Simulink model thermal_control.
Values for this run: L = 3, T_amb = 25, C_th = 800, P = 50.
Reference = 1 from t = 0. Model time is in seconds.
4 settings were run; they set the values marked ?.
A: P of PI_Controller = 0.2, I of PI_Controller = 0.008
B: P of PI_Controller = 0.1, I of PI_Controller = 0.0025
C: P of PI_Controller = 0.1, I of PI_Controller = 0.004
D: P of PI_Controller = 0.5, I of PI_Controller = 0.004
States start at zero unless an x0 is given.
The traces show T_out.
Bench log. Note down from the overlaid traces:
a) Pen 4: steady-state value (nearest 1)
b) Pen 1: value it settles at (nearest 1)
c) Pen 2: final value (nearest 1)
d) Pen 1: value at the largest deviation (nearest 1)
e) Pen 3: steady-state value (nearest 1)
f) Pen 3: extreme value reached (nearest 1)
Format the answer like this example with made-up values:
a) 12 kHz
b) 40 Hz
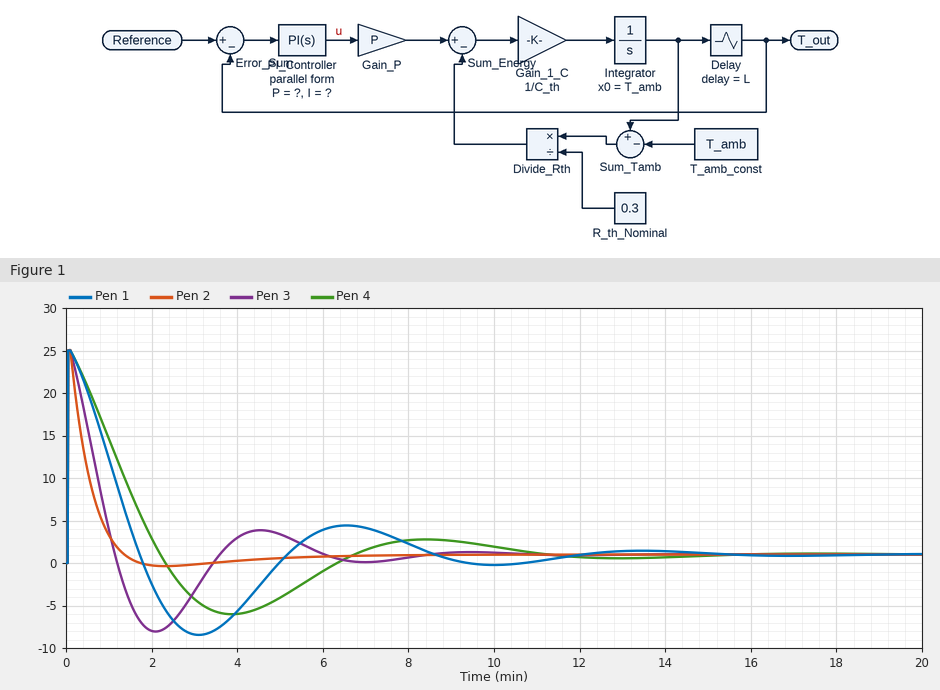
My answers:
a) 1
b) 1
c) 1
d) 25
e) 1
f) 25
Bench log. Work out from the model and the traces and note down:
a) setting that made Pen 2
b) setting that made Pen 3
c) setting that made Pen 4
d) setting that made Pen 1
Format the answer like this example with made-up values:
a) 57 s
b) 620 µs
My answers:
a) D
b) A
c) B
d) C
